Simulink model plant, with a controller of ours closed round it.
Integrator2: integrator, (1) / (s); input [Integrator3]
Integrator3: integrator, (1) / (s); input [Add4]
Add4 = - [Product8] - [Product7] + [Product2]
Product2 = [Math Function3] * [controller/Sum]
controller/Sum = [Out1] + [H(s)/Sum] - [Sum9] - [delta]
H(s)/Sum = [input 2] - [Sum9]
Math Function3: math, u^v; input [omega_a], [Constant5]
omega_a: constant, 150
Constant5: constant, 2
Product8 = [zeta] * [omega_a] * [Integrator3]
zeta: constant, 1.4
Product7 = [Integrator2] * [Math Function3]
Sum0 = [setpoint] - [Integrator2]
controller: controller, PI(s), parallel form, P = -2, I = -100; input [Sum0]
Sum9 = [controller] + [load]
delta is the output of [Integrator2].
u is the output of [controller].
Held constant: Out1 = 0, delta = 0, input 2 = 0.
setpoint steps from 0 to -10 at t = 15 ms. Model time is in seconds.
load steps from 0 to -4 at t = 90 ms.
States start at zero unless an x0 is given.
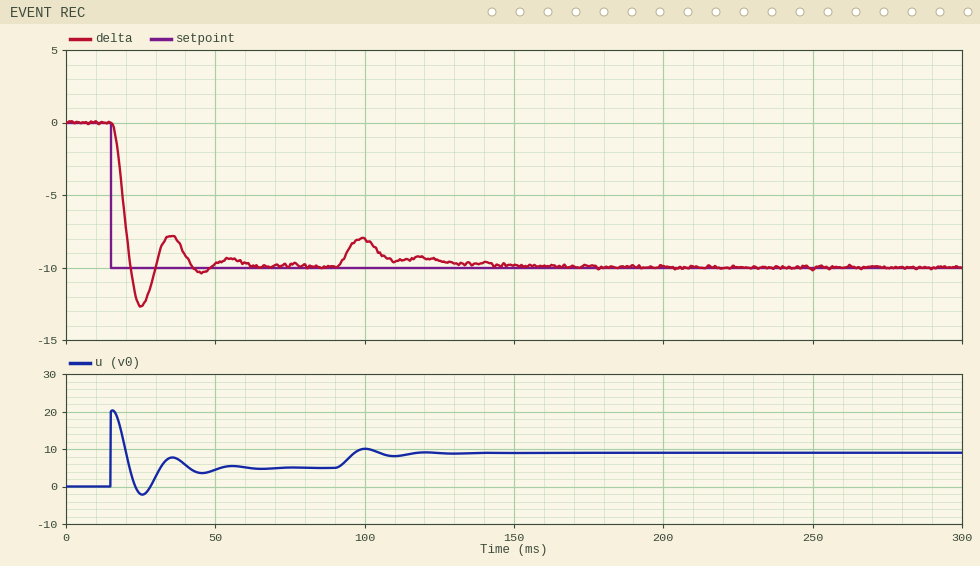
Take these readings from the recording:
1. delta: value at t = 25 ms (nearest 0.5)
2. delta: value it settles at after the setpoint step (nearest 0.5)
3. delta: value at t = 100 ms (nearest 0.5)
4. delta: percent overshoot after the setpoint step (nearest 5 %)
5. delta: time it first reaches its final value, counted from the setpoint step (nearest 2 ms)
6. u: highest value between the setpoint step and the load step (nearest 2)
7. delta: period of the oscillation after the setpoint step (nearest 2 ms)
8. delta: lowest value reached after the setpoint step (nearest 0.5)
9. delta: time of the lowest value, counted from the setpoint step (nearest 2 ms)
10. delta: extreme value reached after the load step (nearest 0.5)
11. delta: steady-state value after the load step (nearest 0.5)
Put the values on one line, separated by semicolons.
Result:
-12.5; -10.0; -8.0; 25 %; 6 ms; 20; 20 ms; -12.5; 10 ms; -8.0; -10.0
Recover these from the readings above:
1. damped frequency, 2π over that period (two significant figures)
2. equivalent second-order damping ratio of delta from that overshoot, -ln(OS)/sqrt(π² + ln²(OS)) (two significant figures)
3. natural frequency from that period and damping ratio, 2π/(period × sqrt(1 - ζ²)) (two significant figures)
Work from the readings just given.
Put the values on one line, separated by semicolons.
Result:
0.31 rad/ms; 0.40; 0.34 rad/ms
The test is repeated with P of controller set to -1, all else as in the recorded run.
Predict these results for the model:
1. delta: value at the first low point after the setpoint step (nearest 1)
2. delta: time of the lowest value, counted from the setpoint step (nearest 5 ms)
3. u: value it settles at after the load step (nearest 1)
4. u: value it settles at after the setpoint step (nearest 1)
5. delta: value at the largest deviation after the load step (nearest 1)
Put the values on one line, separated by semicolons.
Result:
-12; 15 ms; 9; 5; -7
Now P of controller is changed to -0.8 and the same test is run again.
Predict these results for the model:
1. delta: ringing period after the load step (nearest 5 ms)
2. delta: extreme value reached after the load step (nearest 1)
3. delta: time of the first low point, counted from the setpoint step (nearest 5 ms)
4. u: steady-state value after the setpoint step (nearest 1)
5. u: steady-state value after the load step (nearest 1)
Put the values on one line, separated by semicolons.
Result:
30 ms; -7; 15 ms; 5; 9
